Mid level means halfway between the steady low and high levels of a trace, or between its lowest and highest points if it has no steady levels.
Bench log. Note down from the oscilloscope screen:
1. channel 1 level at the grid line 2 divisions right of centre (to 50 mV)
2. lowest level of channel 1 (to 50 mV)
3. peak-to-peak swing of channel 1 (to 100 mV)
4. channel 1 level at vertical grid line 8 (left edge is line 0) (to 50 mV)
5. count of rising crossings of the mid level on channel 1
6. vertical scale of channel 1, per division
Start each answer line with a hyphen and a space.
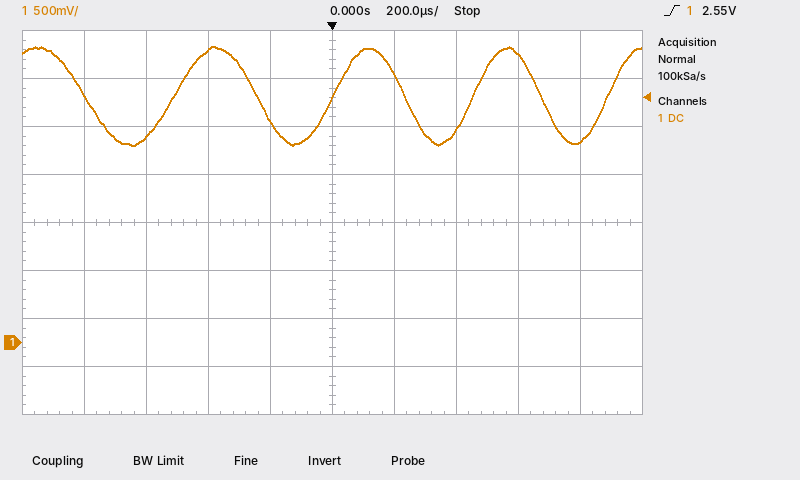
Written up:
- 2.20 V
- 2.05 V
- 1.00 V
- 3.00 V
- 4
- 500 mV
